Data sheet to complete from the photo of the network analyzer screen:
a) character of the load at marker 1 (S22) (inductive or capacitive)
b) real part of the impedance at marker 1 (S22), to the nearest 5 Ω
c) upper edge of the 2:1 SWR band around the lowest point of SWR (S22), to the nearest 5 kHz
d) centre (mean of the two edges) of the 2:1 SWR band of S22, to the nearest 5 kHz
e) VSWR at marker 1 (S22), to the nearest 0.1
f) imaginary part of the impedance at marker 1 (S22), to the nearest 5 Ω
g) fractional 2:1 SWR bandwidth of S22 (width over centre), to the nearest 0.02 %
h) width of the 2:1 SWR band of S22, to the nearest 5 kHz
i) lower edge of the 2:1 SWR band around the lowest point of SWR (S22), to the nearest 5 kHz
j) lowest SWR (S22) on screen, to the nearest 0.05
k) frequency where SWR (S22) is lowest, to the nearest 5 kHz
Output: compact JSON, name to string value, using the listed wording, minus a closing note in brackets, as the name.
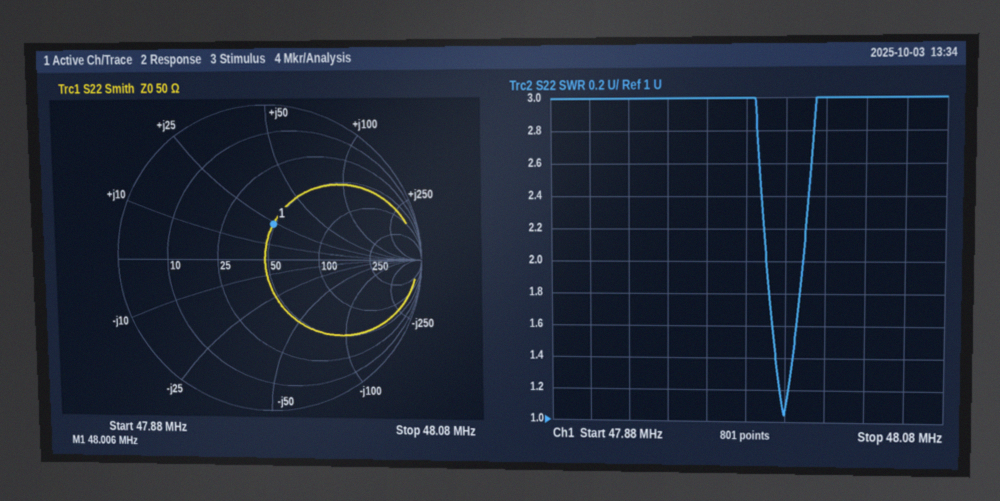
{"character of the load at marker 1 (S22)": "inductive", "real part of the impedance at marker 1 (S22), to the nearest 5 Ω": "50 Ω", "upper edge of the 2:1 SWR band around the lowest point of SWR (S22), to the nearest 5 kHz": "48.010 MHz", "centre (mean of the two edges) of the 2:1 SWR band of S22, to the nearest 5 kHz": "48.000 MHz", "VSWR at marker 1 (S22), to the nearest 0.1": "1.6", "imaginary part of the impedance at marker 1 (S22), to the nearest 5 Ω": "+25 Ω", "fractional 2:1 SWR bandwidth of S22 (width over centre), to the nearest 0.02 %": "0.04 %", "width of the 2:1 SWR band of S22, to the nearest 5 kHz": "20 kHz", "lower edge of the 2:1 SWR band around the lowest point of SWR (S22), to the nearest 5 kHz": "47.990 MHz", "lowest SWR (S22) on screen, to the nearest 0.05": "1.05", "frequency where SWR (S22) is lowest, to the nearest 5 kHz": "48.000 MHz"}
